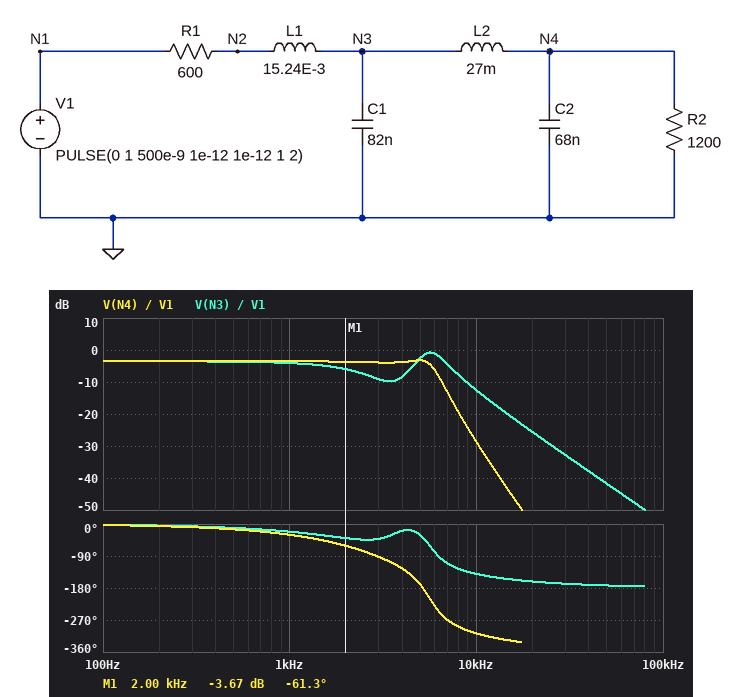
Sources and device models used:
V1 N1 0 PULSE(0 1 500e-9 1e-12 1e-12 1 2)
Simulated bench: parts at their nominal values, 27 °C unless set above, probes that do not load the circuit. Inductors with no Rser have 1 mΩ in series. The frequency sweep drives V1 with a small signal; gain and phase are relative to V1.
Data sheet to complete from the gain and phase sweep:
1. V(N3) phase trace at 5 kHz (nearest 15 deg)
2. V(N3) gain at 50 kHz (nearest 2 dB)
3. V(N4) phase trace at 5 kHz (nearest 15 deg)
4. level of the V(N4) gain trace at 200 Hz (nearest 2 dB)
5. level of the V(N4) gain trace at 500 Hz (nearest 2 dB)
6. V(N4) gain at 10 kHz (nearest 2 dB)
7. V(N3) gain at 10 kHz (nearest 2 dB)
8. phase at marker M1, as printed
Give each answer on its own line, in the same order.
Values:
-30 deg
-42 dB
-165 deg
-4 dB
-4 dB
-28 dB
-12 dB
-61.3 deg
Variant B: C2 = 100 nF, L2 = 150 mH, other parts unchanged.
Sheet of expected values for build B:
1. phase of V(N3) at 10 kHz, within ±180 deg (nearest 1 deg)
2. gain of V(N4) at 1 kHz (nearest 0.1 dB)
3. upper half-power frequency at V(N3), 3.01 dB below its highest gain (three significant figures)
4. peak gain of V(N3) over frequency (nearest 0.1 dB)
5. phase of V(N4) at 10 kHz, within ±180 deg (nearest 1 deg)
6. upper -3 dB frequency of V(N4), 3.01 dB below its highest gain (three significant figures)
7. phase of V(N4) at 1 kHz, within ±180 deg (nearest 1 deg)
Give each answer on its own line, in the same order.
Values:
-142 deg
-3.2 dB
4.89 kHz
0.2 dB
46 deg
1.87 kHz
-66 deg
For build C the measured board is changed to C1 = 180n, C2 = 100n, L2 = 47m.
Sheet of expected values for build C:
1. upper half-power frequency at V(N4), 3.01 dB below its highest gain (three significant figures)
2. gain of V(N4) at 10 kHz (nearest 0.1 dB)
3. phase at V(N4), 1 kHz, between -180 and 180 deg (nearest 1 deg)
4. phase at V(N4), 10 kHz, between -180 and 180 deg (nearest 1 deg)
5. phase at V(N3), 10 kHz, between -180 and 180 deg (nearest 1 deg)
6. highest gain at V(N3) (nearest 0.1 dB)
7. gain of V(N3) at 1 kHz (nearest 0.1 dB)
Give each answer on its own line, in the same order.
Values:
3.30 kHz
-46.2 dB
-51 deg
43 deg
-145 deg
-3.5 dB
-5.4 dB
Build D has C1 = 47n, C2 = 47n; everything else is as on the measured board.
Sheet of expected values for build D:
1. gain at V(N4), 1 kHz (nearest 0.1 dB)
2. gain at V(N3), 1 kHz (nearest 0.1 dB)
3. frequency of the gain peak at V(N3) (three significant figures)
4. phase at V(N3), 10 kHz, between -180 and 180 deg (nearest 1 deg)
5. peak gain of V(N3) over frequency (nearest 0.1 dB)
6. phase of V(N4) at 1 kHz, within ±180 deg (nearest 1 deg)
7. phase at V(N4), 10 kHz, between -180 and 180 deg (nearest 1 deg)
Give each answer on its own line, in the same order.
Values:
-3.4 dB
-3.8 dB
7.46 kHz
-129 deg
1.3 dB
-22 deg
71 deg
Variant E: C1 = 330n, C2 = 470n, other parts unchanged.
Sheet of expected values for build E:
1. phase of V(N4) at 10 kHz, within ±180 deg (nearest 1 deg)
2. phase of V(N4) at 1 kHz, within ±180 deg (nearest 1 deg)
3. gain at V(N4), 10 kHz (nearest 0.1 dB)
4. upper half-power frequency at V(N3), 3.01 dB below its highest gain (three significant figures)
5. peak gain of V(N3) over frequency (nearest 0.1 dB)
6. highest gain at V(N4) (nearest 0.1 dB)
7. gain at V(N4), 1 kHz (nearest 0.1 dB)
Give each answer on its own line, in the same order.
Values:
35 deg
-80 deg
-60.6 dB
2.68 kHz
-1.1 dB
-3.5 dB
-8.4 dB
